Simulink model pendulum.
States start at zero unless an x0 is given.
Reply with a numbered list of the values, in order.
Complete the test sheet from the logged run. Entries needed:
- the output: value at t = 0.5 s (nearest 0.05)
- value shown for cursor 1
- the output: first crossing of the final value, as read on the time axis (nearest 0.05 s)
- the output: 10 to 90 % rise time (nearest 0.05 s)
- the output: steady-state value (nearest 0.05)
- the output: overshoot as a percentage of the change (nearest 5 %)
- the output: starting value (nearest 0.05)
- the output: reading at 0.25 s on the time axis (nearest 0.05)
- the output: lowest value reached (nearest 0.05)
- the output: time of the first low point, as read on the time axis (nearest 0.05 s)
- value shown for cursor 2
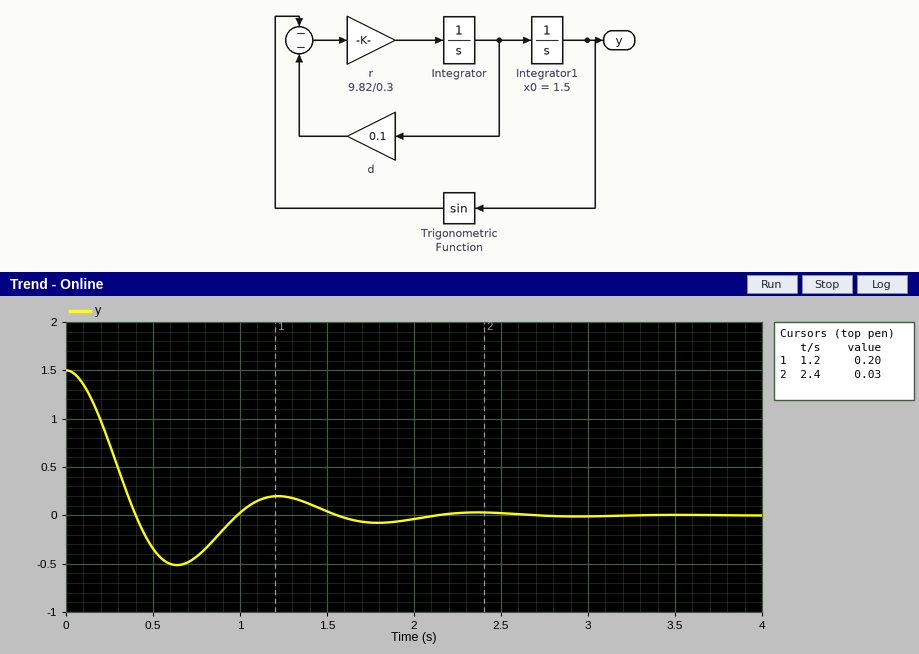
1. -0.35
2. 0.20
3. 0.40 s
4. 0.25 s
5. 0.00
6. 35 %
7. 1.50
8. 0.75
9. -0.50
10. 0.65 s
11. 0.03
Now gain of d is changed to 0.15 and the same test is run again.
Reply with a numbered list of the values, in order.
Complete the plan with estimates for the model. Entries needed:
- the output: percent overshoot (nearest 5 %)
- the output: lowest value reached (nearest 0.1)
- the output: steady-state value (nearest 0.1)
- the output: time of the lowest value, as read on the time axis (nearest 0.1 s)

1. 20 %
2. -0.3
3. 0.0
4. 0.7 s
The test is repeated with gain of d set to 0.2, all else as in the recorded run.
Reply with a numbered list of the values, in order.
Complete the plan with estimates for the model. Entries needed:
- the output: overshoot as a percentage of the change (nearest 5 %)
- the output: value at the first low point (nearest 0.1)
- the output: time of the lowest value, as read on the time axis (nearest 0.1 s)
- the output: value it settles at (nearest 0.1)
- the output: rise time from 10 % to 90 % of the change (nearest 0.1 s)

1. 10 %
2. -0.1
3. 0.8 s
4. 0.0
5. 0.4 s
